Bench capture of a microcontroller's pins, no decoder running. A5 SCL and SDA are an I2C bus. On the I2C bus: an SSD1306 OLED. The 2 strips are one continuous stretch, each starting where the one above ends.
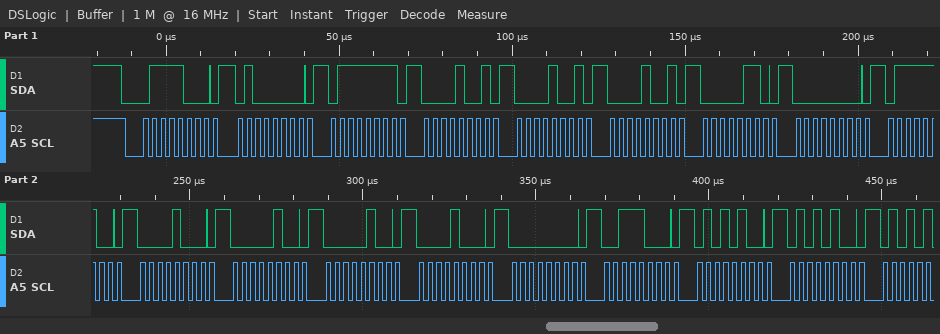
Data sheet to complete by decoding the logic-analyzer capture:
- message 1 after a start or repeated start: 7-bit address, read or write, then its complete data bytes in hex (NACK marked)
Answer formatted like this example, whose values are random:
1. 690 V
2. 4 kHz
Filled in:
1. 0x3C write: 40 7F 09 09 09 06 00 7C 08 04 04 08 00 38 54 54
